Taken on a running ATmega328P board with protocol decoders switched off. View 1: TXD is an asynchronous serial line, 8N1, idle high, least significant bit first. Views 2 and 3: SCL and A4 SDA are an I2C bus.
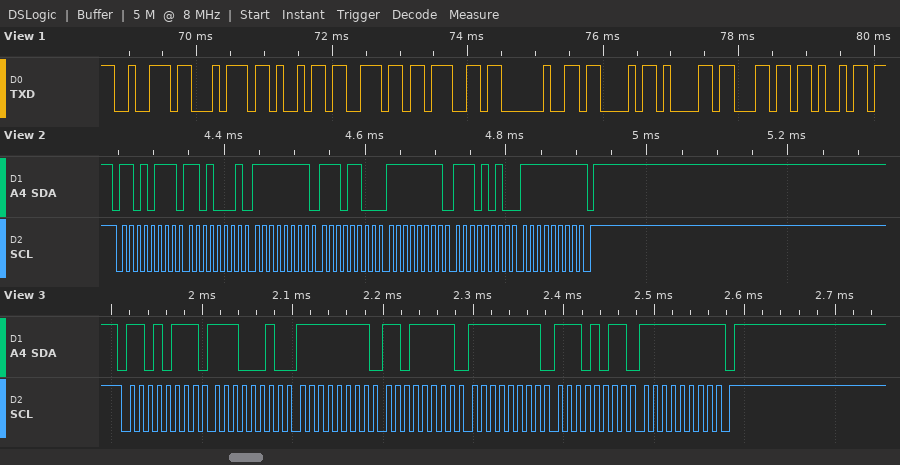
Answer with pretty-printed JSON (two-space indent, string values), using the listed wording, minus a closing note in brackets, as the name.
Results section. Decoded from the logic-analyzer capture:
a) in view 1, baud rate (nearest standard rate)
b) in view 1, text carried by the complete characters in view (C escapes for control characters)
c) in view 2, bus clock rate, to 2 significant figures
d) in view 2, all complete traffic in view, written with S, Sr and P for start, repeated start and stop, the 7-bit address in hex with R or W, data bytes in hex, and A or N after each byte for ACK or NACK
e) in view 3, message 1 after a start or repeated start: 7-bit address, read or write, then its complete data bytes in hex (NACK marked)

{
  "in view 1, baud rate": "9600 baud",
  "in view 1, text carried by the complete characters in view": "\"rting Cali\"",
  "in view 2, bus clock rate, to 2 significant figures": "100 kHz",
  "in view 2, all complete traffic in view, written with S, Sr and P for start, repeated start and stop, the 7-bit address in hex with R or W, data bytes in hex, and A or N after each byte for ACK or NACK": "S 6BR A D1 A FF A EC A FF A EA A FF N P",
  "in view 3, message 1 after a start or repeated start: 7-bit address, read or write, then its complete data bytes in hex": "0x6B read: E2 FF DF FF EB FF NACK"
}
